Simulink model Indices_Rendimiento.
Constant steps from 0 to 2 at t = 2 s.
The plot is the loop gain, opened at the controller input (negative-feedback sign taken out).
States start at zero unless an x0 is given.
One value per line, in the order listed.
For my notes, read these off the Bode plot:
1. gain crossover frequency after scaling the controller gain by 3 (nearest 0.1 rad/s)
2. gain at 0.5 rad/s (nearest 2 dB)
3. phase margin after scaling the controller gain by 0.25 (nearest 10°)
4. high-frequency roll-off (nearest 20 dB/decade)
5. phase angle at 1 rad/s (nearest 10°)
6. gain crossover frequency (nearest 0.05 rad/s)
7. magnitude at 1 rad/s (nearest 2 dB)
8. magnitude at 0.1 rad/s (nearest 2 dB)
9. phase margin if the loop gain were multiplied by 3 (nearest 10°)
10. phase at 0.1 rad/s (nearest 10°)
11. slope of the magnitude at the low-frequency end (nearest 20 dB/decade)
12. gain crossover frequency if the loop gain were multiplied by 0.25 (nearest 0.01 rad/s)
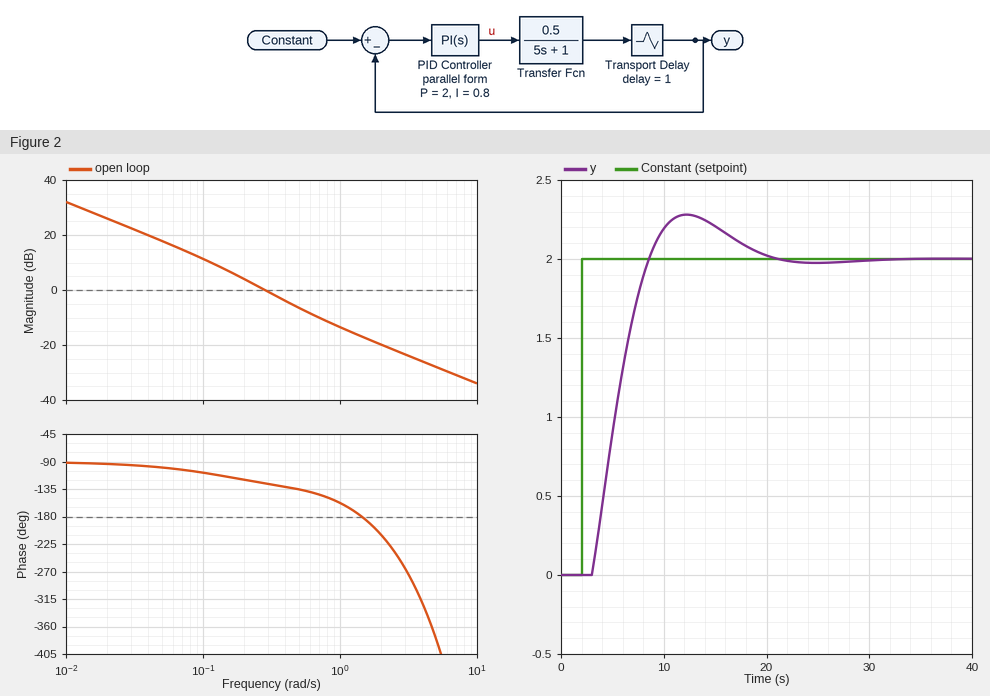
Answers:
0.7 rad/s
-6 dB
70°
-20 dB/decade
-160°
0.30 rad/s
-14 dB
12 dB
40°
-110°
-20 dB/decade
0.09 rad/s
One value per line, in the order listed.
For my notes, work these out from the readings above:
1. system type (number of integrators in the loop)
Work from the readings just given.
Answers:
1
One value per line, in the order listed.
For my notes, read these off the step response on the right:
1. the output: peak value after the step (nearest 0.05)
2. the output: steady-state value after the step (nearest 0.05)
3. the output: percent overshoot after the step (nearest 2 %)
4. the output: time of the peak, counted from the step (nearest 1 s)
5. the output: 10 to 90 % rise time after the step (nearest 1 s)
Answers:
2.30
2.00
14 %
10 s
4 s
